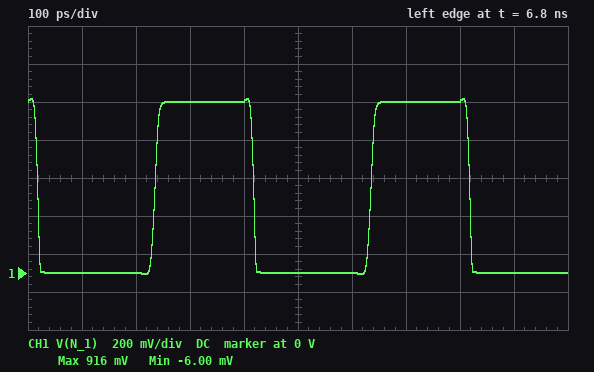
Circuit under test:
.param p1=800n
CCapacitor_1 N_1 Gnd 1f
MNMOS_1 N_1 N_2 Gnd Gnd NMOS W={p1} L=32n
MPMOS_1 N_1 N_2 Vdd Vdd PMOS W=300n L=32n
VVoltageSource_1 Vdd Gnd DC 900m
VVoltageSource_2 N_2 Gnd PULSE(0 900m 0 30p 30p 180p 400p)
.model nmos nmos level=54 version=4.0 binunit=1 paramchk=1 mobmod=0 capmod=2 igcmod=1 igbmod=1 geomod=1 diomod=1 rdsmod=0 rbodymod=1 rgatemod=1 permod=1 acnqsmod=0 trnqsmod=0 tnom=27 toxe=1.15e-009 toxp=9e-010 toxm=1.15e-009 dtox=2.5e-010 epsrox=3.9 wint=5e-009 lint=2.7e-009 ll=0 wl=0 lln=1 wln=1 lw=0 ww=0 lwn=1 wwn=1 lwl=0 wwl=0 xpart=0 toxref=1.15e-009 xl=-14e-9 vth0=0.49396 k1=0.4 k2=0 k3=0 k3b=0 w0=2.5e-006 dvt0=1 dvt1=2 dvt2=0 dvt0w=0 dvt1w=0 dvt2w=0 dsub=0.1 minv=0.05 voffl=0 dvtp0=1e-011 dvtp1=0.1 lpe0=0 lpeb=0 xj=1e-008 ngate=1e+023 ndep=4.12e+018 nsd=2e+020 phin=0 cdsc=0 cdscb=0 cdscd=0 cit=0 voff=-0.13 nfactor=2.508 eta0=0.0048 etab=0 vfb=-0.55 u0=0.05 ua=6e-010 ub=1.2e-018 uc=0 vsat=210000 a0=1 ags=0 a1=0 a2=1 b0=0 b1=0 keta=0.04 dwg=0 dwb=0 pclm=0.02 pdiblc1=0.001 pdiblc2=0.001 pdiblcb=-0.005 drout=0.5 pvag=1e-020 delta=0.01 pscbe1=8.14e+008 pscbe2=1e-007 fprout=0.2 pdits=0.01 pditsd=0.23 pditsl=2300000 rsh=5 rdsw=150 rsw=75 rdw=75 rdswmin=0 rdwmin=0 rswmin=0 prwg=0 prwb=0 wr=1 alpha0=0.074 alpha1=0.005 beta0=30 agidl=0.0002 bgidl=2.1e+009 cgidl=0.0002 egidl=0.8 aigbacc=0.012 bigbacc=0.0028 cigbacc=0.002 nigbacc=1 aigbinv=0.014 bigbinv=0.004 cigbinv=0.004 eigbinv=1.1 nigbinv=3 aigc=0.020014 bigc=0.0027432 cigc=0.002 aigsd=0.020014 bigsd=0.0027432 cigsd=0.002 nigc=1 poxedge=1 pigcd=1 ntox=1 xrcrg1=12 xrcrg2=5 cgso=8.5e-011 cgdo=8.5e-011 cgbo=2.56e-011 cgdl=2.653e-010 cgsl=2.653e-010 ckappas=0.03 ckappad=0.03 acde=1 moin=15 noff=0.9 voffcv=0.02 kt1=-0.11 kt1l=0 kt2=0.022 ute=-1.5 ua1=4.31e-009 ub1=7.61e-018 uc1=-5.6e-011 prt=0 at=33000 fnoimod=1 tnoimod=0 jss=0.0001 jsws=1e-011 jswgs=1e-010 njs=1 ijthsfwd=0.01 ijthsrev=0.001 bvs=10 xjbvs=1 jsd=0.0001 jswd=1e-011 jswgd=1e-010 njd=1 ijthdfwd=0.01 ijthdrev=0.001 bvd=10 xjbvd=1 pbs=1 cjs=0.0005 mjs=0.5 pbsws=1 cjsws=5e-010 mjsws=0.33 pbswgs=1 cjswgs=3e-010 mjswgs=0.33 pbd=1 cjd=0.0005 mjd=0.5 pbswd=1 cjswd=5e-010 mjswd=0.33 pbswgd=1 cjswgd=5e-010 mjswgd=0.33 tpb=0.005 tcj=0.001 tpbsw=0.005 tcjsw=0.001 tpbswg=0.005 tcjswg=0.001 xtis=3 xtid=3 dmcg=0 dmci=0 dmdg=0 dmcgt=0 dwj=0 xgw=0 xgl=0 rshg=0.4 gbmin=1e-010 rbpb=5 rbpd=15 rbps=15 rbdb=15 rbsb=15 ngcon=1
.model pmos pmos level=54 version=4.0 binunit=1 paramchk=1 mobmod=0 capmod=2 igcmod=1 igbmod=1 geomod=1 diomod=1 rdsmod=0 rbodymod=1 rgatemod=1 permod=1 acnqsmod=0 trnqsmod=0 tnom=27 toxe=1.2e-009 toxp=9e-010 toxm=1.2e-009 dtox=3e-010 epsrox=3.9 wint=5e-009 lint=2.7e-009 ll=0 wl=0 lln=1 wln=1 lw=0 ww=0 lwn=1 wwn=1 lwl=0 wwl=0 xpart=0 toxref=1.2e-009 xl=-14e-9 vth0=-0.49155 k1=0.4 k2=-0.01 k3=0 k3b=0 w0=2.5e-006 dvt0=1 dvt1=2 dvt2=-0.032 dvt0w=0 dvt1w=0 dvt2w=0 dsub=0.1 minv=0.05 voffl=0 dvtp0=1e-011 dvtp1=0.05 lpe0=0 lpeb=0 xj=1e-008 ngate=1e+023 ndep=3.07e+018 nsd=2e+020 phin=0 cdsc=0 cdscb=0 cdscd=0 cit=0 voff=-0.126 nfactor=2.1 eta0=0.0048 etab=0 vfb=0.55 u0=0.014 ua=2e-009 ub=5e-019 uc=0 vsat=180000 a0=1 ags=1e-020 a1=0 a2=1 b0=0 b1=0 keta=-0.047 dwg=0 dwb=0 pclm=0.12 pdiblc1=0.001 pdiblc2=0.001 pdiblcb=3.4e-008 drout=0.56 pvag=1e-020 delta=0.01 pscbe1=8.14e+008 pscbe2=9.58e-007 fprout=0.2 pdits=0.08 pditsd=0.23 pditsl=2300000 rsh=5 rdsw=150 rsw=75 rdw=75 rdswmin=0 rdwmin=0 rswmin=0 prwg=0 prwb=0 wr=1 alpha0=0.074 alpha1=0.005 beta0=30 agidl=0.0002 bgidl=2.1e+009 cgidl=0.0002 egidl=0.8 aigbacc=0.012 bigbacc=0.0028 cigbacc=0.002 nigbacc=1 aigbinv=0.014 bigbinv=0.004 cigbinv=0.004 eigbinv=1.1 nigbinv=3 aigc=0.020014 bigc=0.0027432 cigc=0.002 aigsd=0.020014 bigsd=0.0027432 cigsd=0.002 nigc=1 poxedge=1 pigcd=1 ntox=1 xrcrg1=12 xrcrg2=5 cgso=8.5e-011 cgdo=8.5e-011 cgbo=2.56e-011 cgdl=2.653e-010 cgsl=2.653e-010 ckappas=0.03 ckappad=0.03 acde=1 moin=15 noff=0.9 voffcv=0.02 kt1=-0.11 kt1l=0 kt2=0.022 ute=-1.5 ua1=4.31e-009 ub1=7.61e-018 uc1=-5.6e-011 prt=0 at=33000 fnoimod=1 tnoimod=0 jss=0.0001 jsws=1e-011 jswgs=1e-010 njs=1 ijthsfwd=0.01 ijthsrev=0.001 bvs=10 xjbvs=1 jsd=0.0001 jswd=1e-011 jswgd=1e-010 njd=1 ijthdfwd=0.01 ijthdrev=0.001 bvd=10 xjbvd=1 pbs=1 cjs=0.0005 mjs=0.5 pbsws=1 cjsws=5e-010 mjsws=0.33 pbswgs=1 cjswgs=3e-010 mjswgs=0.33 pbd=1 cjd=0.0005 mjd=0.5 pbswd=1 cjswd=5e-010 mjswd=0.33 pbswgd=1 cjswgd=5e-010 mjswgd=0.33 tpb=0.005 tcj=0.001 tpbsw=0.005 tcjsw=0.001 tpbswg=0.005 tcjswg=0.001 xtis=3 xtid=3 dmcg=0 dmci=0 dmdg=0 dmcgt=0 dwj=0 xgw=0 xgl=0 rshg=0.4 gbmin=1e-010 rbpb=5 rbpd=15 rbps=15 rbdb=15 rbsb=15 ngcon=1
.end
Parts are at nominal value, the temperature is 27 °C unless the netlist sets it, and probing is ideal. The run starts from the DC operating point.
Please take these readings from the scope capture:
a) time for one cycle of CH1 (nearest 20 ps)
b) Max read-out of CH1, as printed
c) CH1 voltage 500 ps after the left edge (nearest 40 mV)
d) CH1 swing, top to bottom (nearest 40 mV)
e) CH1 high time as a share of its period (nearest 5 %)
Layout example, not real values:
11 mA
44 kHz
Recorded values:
400 ps
916 mV
0 V
920 mV
45 %
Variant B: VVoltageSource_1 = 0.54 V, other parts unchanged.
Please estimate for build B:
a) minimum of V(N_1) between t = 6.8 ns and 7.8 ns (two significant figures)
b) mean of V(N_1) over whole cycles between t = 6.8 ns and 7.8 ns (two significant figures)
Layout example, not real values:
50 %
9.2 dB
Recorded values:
-59 mV
210 mV
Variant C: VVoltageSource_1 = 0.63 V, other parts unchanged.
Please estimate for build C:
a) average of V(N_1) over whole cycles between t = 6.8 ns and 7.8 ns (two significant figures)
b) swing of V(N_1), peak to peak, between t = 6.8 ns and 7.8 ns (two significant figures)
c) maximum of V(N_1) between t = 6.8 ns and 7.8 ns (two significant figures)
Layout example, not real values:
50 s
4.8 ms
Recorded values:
270 mV
700 mV
670 mV
